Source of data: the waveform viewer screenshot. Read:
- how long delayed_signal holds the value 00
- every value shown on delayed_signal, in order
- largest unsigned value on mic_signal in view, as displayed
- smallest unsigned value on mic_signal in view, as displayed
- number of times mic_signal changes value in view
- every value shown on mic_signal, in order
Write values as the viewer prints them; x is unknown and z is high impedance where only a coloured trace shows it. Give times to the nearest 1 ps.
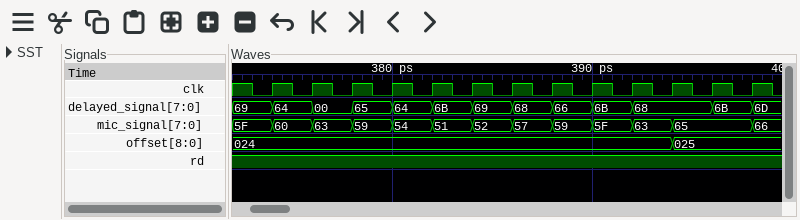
2 ps
69, 64, 00, 65, 64, 6B, 69, 68, 66, 6B, 68, 6B, 6D
66
51
12
5F, 60, 63, 59, 54, 51, 52, 57, 59, 5F, 63, 65, 66
